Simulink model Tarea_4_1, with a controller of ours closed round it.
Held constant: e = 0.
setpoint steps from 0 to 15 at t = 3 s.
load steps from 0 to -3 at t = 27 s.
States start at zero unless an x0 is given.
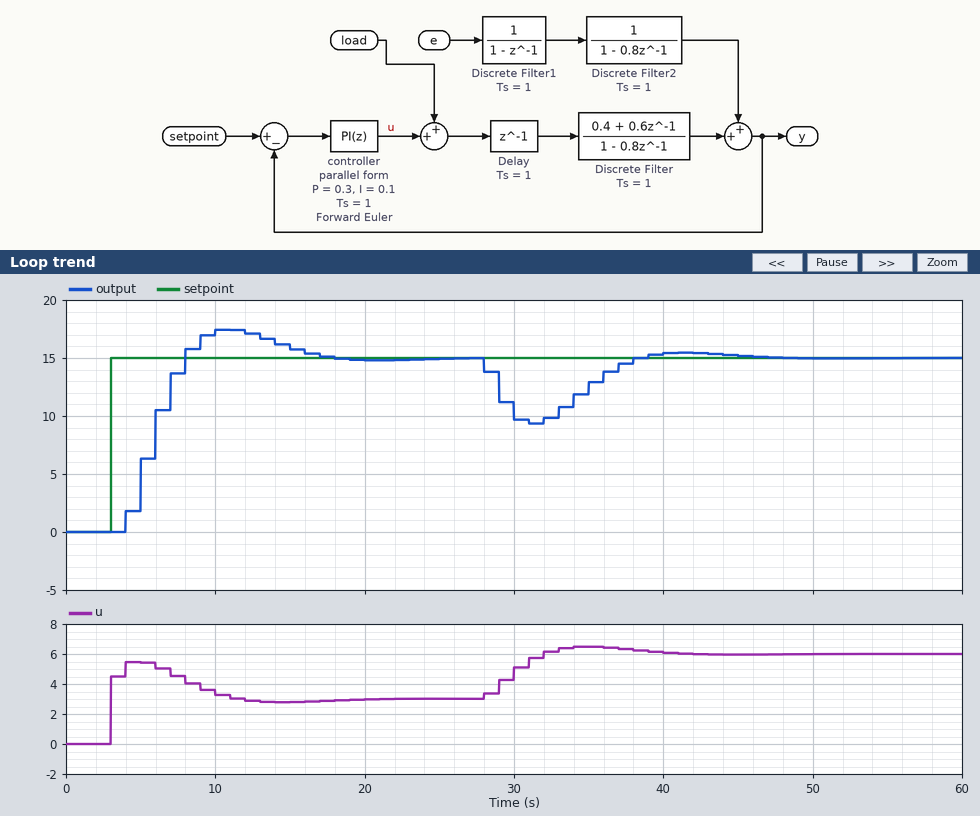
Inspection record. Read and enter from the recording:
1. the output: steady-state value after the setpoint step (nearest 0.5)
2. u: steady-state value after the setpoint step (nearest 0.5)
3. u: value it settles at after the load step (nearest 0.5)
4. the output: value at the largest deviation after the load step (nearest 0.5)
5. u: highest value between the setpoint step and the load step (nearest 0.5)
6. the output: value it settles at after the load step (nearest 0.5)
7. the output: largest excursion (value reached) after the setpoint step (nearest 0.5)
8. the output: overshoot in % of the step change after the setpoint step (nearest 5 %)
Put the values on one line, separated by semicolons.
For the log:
15.0; 3.0; 6.0; 9.5; 5.5; 15.0; 17.5; 15 %
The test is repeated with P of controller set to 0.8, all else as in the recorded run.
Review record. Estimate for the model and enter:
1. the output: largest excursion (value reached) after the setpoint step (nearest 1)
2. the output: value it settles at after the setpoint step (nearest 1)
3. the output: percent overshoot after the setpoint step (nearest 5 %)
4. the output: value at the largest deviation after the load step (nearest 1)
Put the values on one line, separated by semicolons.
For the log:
19; 15; 25 %; 11
